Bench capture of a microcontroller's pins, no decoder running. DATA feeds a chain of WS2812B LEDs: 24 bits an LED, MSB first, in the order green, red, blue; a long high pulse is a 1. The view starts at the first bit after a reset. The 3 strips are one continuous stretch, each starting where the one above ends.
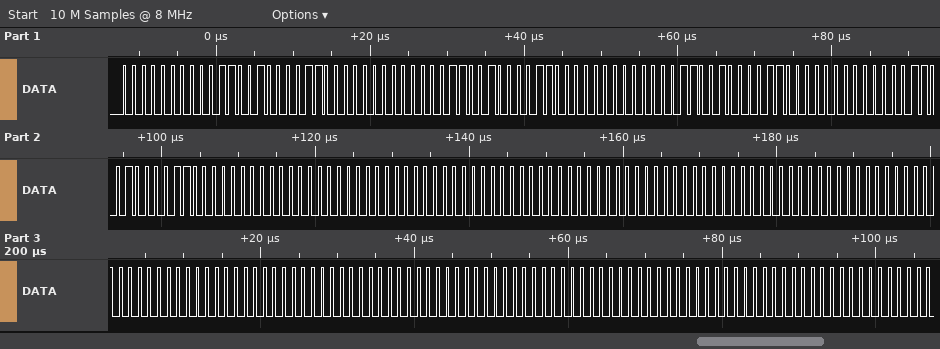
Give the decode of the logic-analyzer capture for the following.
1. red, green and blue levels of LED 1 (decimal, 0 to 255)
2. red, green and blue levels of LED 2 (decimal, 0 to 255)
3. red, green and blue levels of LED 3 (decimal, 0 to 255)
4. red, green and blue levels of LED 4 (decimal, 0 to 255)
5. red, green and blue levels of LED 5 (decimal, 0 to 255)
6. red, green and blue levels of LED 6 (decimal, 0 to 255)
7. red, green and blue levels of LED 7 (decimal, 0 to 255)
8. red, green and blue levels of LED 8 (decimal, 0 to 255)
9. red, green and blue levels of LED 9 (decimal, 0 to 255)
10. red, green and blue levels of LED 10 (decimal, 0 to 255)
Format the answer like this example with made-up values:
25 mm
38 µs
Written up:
50, 0, 24
50, 0, 24
50, 0, 24
50, 0, 24
0, 0, 0
0, 0, 0
0, 0, 0
0, 0, 0
0, 0, 0
0, 0, 0
